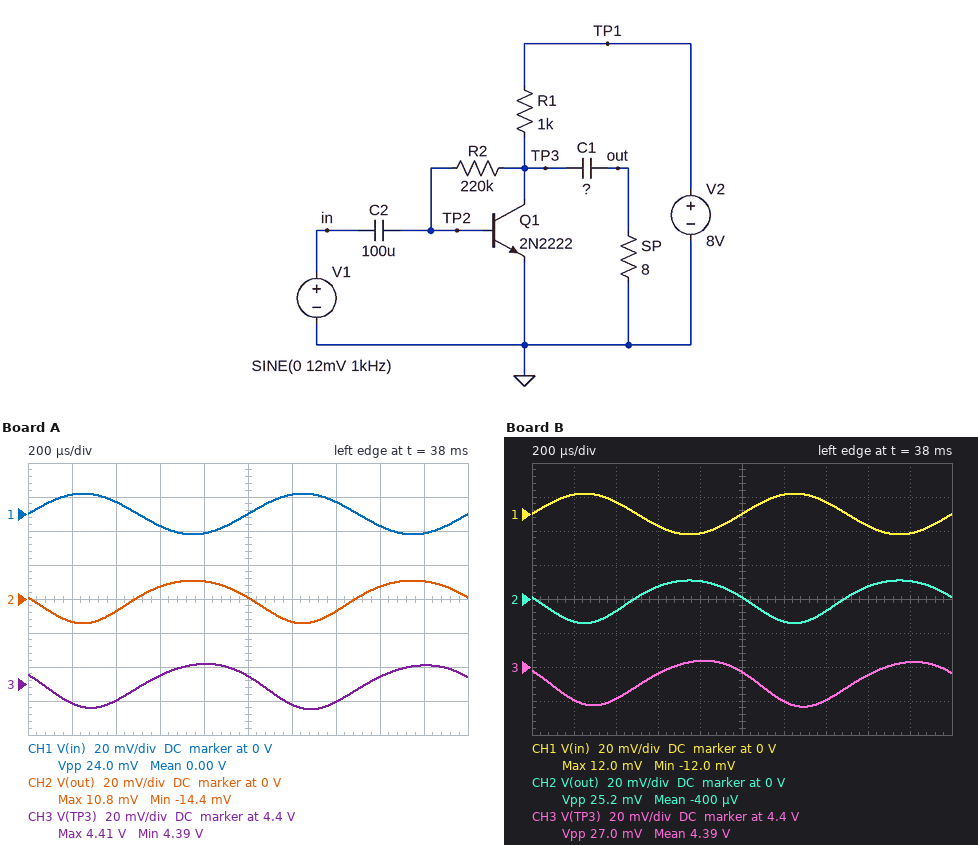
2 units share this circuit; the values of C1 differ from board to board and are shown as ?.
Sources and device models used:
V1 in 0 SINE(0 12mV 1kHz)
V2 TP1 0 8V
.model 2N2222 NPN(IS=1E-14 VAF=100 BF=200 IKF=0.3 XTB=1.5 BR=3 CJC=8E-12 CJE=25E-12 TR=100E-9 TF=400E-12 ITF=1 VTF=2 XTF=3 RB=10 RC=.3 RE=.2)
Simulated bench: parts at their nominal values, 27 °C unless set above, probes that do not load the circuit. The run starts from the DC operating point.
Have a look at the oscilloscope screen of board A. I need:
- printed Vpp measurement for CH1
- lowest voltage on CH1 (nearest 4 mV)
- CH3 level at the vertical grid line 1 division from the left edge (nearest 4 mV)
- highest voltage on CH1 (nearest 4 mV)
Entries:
24.0 mV
-12 mV
4.388 V
12 mV
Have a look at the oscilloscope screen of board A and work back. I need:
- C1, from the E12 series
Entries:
68 µF
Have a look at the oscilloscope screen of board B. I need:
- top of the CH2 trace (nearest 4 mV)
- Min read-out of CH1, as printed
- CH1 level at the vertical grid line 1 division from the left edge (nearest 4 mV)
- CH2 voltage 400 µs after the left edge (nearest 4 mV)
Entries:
12 mV
-12.0 mV
12 mV
-8 mV
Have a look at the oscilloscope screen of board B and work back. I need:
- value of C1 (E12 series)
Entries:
56 µF
